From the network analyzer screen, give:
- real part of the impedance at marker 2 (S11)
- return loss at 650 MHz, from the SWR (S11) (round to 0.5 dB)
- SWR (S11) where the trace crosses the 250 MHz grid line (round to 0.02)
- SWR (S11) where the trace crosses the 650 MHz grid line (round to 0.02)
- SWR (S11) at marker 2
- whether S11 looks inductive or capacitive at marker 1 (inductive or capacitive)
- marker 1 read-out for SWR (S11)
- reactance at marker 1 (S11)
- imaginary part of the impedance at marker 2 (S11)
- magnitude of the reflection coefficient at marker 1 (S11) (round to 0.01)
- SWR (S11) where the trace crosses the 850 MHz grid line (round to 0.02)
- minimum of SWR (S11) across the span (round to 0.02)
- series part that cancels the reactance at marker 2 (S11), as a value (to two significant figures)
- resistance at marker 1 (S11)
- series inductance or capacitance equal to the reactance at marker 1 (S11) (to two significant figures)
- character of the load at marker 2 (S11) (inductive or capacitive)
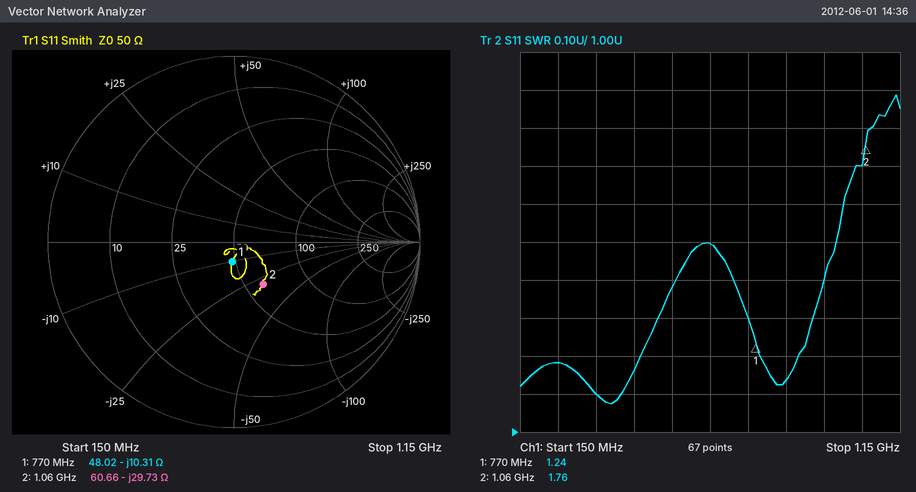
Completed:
60.66 Ω
14.0 dB
1.18
1.50
1.76
capacitive
1.24
-10.31 Ω
-29.73 Ω
0.11
1.14
1.08
4.5 nH
48.02 Ω
20 pF
capacitive
